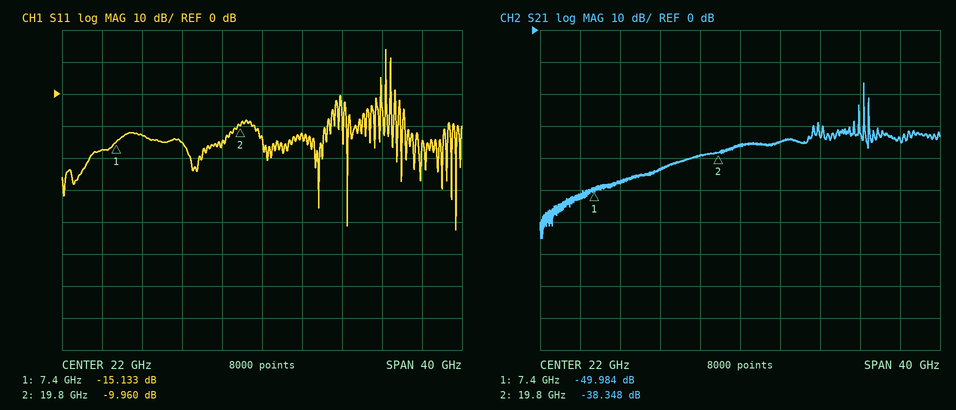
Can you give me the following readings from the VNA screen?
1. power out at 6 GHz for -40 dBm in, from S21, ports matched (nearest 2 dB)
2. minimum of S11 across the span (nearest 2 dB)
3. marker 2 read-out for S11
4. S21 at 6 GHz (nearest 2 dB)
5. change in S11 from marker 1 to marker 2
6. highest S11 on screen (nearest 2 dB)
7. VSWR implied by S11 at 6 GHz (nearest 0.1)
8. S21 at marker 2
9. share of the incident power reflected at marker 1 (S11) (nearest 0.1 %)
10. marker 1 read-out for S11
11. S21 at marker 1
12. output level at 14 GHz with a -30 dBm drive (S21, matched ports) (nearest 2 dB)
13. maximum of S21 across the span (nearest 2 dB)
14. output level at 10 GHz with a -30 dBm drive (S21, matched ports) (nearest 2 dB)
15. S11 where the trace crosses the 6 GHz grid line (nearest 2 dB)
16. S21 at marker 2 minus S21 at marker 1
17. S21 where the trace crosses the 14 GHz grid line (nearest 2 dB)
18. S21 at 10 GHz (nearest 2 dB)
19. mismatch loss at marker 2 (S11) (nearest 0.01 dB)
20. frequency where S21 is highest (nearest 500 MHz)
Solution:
-92 dBm
-42 dB
-9.960 dB
-52 dB
5.173 dB
14 dB
1.3
-38.348 dB
3.1 %
-15.133 dB
-49.984 dB
-74 dBm
-16 dB
-78 dBm
-18 dB
11.636 dB
-44 dB
-48 dB
0.46 dB
34.5 GHz
